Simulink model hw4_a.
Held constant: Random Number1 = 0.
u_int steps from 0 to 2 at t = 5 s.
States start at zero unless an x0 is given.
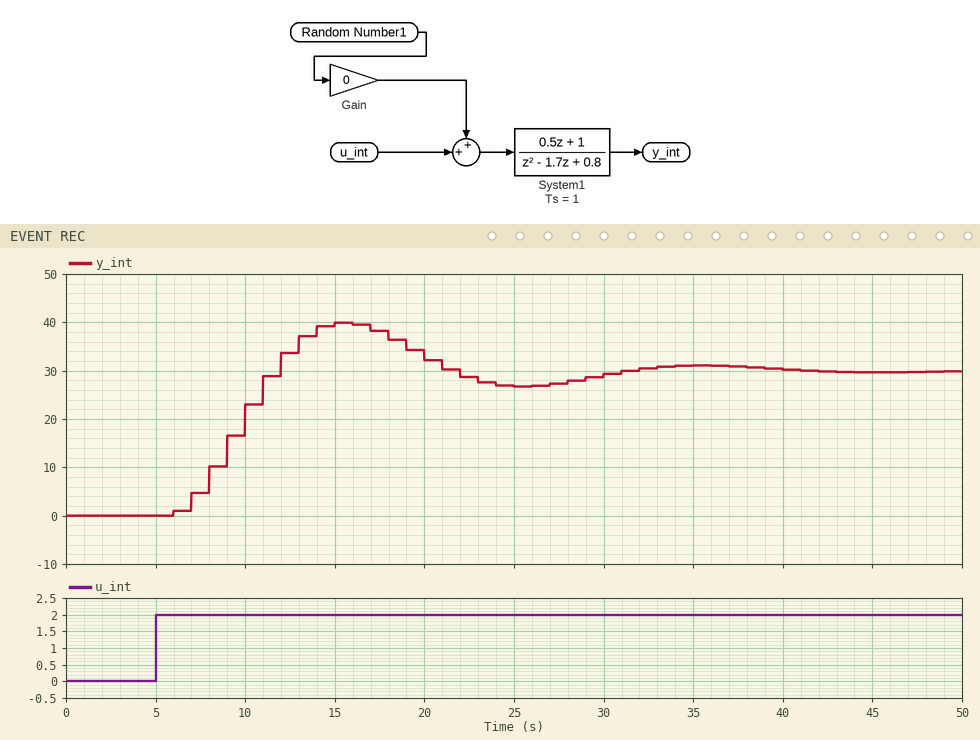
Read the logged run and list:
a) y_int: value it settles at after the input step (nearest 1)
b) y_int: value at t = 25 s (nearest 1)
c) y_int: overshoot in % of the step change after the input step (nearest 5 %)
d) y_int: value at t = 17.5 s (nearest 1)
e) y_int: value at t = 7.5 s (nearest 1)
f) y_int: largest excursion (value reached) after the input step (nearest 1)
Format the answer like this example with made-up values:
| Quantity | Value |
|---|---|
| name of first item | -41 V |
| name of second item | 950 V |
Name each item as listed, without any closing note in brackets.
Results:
| Quantity | Value |
|---|---|
| y_int: value it settles at after the input step | 30 |
| y_int: value at t = 25 s | 27 |
| y_int: overshoot in % of the step change after the input step | 35 % |
| y_int: value at t = 17.5 s | 38 |
| y_int: value at t = 7.5 s | 5 |
| y_int: largest excursion (value reached) after the input step | 40 |
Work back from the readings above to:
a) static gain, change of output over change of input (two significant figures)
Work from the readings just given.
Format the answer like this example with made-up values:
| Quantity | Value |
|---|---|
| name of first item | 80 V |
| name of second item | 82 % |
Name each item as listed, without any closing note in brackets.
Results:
| Quantity | Value |
|---|---|
| static gain, change of output over change of input | 15 |
